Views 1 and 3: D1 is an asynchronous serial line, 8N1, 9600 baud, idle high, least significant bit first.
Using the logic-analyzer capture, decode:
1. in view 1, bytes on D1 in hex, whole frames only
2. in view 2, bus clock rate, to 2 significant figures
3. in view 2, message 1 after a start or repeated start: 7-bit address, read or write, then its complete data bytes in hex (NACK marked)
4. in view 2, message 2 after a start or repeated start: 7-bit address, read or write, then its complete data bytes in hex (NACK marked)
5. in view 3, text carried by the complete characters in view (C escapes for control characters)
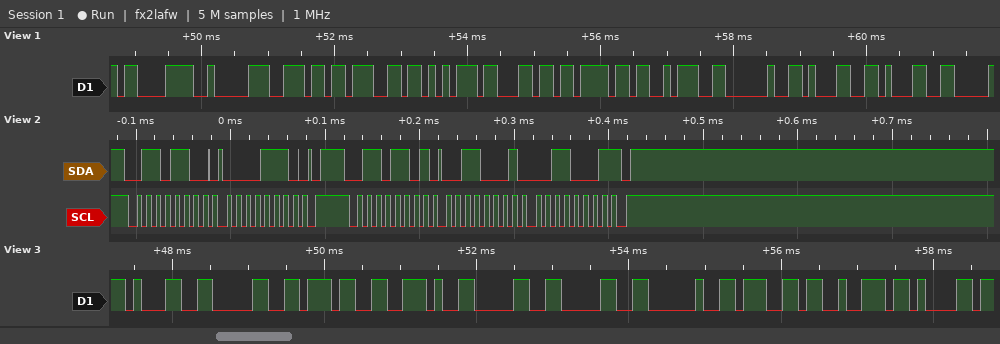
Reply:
0xC3 0x82 0x6E 0x67 0x75 0x6C 0x6F 0x3A 0x20 0x31 0x31
100 kHz
0x36 write: 0E
0x36 read: 31 31 NACK
"107.00 gra"
